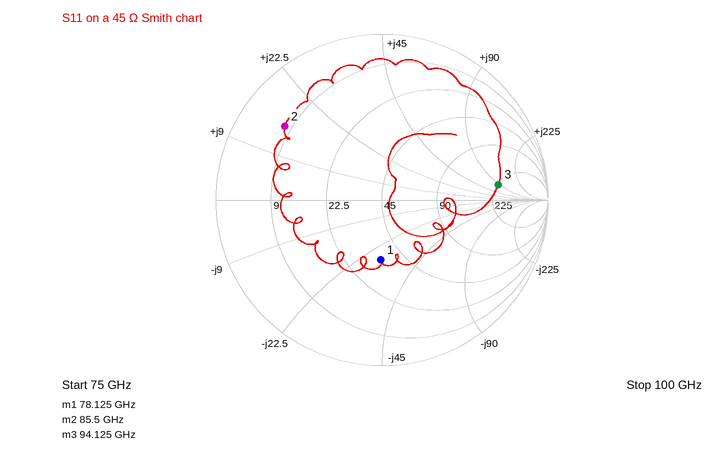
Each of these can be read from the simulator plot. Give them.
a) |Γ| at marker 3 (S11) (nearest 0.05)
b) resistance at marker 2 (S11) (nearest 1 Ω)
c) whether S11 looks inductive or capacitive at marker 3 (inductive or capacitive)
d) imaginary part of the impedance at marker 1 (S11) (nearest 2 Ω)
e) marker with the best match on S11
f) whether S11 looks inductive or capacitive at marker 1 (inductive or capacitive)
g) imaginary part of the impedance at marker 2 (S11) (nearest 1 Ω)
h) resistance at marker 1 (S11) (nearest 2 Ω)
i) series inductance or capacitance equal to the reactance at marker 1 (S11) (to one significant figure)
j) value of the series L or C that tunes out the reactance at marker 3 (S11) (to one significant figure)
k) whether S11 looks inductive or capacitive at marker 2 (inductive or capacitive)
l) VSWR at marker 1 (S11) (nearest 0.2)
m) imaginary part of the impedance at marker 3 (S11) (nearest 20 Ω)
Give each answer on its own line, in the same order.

0.70
8 Ω
inductive
-28 Ω
marker 1
capacitive
+15 Ω
34 Ω
70 fF
20 fF
inductive
2.2
+80 Ω
